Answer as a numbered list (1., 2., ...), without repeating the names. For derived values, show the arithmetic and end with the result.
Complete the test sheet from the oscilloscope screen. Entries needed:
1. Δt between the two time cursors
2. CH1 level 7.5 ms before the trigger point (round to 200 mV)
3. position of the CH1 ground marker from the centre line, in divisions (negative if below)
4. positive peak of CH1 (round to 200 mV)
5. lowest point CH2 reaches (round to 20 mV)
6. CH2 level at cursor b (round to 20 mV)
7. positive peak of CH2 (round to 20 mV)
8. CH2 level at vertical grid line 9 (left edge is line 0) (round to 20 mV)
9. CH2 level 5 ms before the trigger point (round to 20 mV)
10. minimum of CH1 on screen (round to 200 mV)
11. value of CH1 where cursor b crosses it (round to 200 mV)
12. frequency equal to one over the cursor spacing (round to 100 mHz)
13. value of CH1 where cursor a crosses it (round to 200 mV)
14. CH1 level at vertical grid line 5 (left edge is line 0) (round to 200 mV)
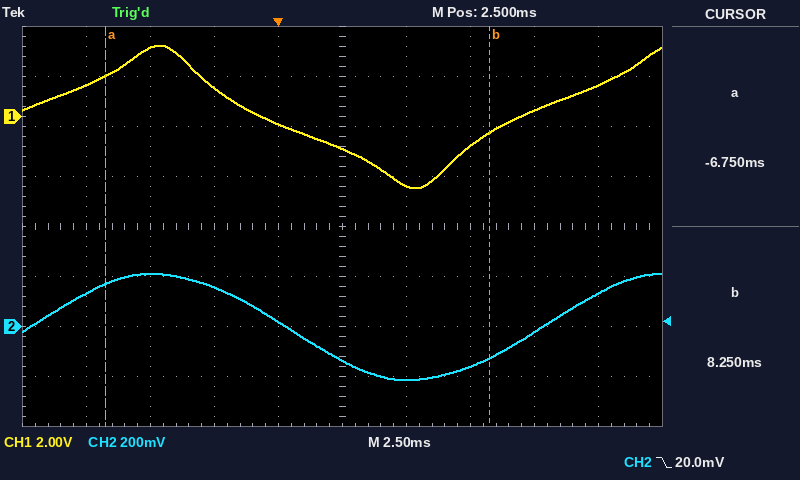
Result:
1. 8.25 ms − (-6.75 ms) = 15.00 ms
2. 1.2 V
3. +2.2 div
4. 2.8 V
5. -220 mV
6. -120 mV
7. 220 mV
8. 140 mV
9. 220 mV
10. -2.8 V
11. -600 mV
12. 1 / 15.00 ms ≈ 66.7 Hz
13. 1.6 V
14. -1.2 V
